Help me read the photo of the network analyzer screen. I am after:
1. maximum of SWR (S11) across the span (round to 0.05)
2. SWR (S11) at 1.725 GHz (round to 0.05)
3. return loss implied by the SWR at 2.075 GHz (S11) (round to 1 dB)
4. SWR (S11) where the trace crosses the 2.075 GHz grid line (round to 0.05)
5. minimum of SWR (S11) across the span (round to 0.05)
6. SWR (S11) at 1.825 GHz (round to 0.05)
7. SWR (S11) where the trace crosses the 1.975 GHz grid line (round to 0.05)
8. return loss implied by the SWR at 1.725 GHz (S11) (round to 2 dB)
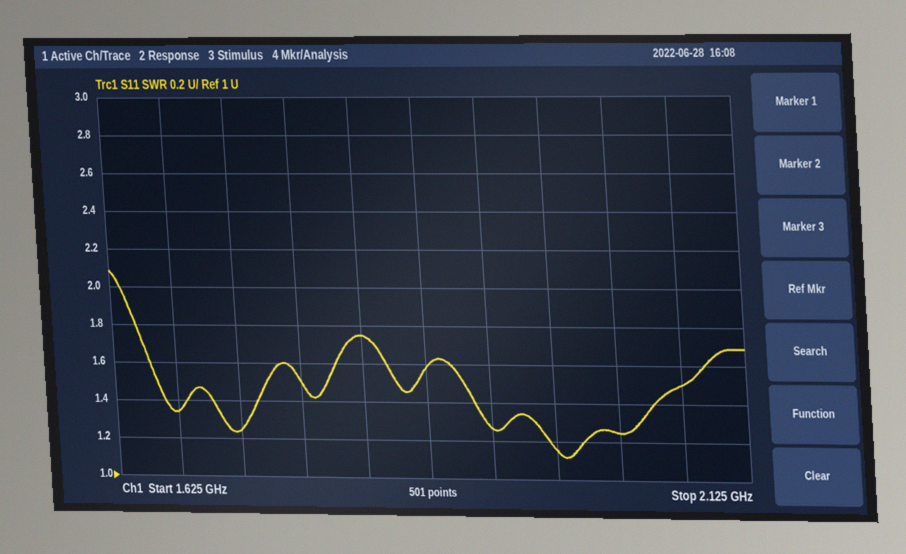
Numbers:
2.10
1.25
14 dB
1.50
1.10
1.75
1.15
20 dB
